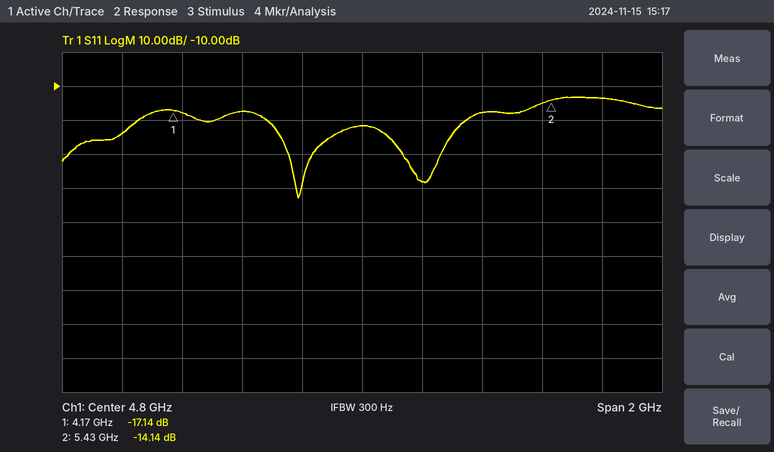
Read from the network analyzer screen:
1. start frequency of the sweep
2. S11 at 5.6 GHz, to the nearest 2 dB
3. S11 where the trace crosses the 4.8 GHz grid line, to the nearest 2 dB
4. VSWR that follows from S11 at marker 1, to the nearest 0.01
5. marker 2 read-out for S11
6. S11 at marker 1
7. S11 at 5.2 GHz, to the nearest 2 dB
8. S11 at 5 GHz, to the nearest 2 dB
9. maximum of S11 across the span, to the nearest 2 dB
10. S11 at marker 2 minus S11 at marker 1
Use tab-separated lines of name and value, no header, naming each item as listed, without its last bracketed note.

start frequency of the sweep	3.8 GHz
S11 at 5.6 GHz, to the nearest 2 dB	-14 dB
S11 where the trace crosses the 4.8 GHz grid line, to the nearest 2 dB	-22 dB
VSWR that follows from S11 at marker 1, to the nearest 0.01	1.32
marker 2 read-out for S11	-14.14 dB
S11 at marker 1	-17.14 dB
S11 at 5.2 GHz, to the nearest 2 dB	-18 dB
S11 at 5 GHz, to the nearest 2 dB	-38 dB
maximum of S11 across the span, to the nearest 2 dB	-14 dB
S11 at marker 2 minus S11 at marker 1	3.00 dB
